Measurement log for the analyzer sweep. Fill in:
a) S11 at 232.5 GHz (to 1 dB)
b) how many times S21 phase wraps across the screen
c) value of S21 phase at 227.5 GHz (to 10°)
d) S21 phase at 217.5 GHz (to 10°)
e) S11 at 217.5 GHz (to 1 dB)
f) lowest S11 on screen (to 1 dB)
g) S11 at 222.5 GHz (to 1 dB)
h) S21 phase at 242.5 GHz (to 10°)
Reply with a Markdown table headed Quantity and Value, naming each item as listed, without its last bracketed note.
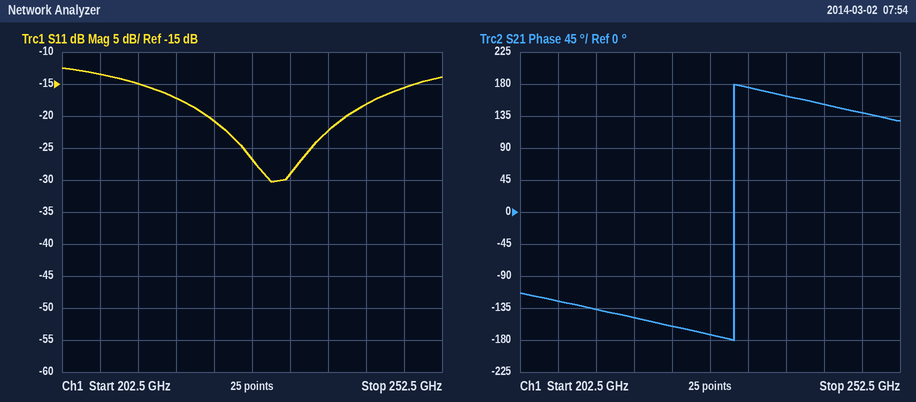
| Quantity | Value |
|---|---|
| S11 at 232.5 GHz | -29 dB |
| how many times S21 phase wraps across the screen | 1 |
| value of S21 phase at 227.5 GHz | -170° |
| S21 phase at 217.5 GHz | -150° |
| S11 at 217.5 GHz | -17 dB |
| lowest S11 on screen | -30 dB |
| S11 at 222.5 GHz | -21 dB |
| S21 phase at 242.5 GHz | 150° |
